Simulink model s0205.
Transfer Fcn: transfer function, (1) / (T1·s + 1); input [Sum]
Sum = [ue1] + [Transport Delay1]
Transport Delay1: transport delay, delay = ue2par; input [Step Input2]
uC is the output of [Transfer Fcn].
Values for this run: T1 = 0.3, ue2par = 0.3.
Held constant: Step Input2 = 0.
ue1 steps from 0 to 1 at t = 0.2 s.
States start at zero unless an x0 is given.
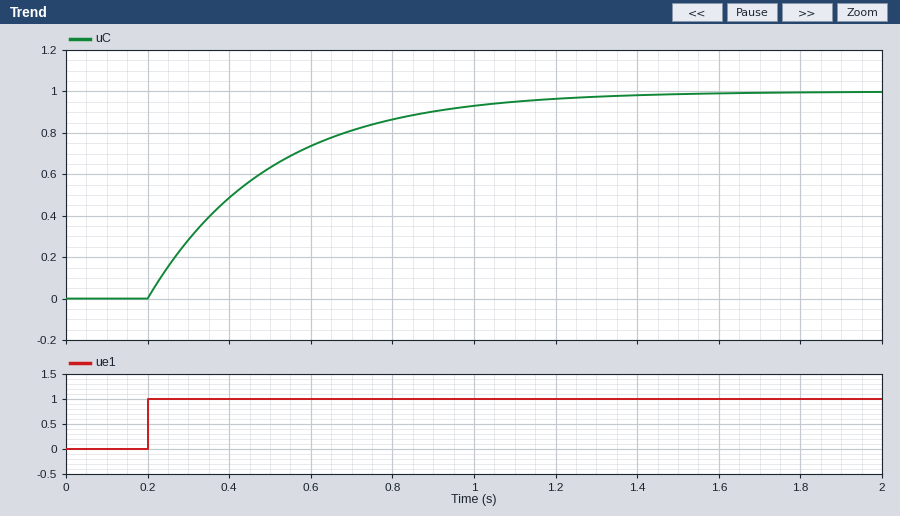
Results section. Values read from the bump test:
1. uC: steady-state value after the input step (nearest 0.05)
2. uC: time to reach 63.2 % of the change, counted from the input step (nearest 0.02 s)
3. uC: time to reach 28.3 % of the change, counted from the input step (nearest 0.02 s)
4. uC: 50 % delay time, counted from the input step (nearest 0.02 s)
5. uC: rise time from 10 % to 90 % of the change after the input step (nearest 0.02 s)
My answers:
1.00
0.30 s
0.10 s
0.20 s
0.66 s
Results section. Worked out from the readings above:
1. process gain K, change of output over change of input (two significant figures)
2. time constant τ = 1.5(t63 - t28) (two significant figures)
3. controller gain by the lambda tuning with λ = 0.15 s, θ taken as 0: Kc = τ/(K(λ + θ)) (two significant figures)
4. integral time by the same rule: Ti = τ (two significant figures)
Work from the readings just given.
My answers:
1.0
0.30 s
2.0
0.30 s
